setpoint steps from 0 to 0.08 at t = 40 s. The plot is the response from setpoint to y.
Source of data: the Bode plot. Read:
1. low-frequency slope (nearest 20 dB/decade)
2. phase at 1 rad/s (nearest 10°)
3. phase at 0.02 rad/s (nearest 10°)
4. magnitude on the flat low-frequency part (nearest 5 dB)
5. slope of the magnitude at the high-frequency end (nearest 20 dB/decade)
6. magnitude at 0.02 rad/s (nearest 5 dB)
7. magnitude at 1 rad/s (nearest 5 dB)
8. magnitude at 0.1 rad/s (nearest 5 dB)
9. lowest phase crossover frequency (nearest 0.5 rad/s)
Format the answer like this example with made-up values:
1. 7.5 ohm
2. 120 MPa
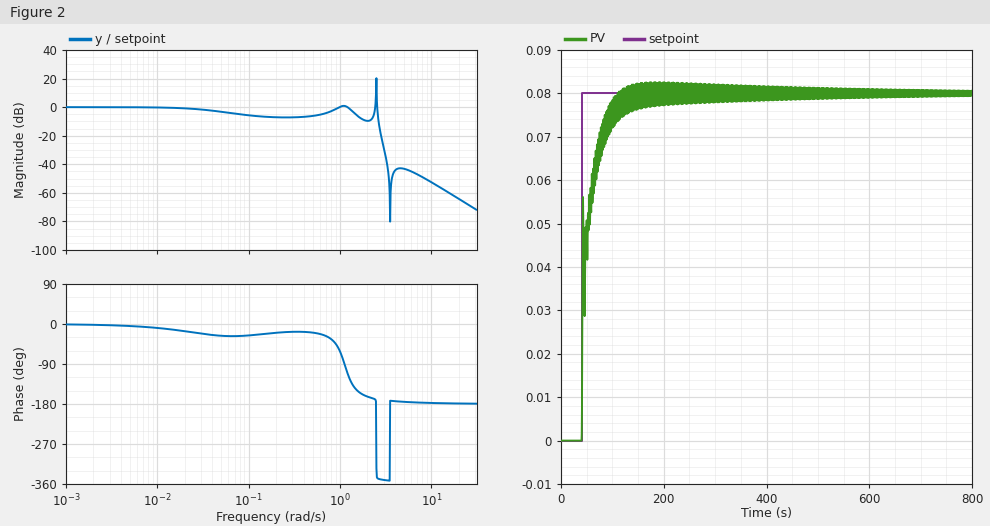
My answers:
1. 0 dB/decade
2. -60°
3. -20°
4. 0 dB
5. -40 dB/decade
6. 0 dB
7. 0 dB
8. -5 dB
9. 2.5 rad/s
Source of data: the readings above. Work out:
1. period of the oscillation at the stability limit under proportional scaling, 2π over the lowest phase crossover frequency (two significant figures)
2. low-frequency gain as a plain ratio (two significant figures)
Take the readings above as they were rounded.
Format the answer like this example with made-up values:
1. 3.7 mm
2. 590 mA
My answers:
1. 2.5 s
2. 1.0
